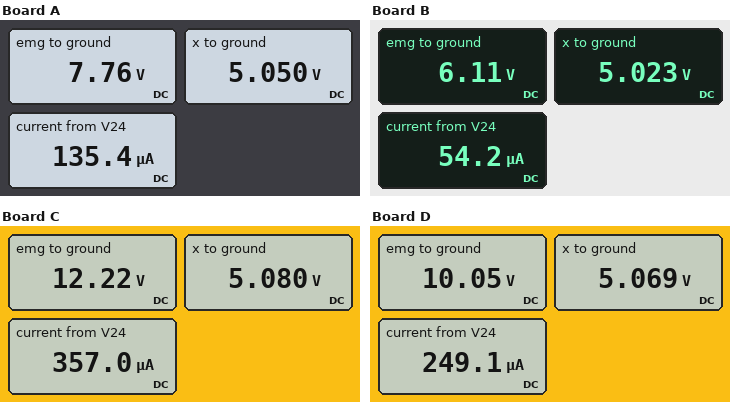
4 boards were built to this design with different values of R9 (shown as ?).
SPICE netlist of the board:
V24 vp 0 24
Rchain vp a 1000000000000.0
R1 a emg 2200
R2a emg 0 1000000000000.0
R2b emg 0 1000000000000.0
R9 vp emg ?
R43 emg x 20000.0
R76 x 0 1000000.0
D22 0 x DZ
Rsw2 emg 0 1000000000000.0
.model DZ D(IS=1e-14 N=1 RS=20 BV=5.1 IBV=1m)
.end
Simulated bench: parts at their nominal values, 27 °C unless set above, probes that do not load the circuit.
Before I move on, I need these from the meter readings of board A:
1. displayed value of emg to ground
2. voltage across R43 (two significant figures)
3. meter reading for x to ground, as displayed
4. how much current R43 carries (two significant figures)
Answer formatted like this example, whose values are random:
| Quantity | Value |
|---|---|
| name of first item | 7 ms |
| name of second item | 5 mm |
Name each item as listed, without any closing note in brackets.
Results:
| Quantity | Value |
|---|---|
| displayed value of emg to ground | 7.76 V |
| voltage across R43 | 2.7 V |
| meter reading for x to ground, as displayed | 5.050 V |
| how much current R43 carries | 140 µA |
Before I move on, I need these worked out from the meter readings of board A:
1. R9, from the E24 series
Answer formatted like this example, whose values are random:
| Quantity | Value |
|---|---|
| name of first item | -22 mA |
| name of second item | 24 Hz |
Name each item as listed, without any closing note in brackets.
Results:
| Quantity | Value |
|---|---|
| R9, from the E24 series | 120 kΩ |
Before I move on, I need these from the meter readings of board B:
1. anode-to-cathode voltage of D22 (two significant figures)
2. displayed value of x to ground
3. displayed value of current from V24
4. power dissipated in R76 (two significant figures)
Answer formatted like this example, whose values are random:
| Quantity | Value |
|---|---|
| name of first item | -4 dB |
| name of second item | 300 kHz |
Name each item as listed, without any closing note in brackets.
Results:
| Quantity | Value |
|---|---|
| anode-to-cathode voltage of D22 | -5.0 V |
| displayed value of x to ground | 5.023 V |
| displayed value of current from V24 | 54.2 µA |
| power dissipated in R76 | 25 µW |
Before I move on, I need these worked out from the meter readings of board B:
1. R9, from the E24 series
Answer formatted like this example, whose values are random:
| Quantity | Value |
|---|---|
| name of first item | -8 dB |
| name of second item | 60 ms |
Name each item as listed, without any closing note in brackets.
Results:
| Quantity | Value |
|---|---|
| R9, from the E24 series | 330 kΩ |
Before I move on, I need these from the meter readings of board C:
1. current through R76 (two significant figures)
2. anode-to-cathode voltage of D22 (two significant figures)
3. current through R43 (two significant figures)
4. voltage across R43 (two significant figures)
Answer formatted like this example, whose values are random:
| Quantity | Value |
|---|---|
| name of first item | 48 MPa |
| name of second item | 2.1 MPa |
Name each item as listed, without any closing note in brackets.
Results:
| Quantity | Value |
|---|---|
| current through R76 | 5.1 µA |
| anode-to-cathode voltage of D22 | -5.1 V |
| current through R43 | 360 µA |
| voltage across R43 | 7.1 V |
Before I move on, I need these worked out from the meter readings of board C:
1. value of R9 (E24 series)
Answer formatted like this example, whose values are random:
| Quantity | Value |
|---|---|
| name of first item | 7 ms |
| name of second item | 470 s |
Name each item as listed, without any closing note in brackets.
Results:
| Quantity | Value |
|---|---|
| value of R9 | 33 kΩ |
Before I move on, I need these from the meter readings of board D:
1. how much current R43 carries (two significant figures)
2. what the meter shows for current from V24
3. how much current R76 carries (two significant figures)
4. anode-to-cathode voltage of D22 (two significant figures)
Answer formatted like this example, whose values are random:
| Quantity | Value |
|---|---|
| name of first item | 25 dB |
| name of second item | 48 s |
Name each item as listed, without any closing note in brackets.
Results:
| Quantity | Value |
|---|---|
| how much current R43 carries | 250 µA |
| what the meter shows for current from V24 | 249.1 µA |
| how much current R76 carries | 5.1 µA |
| anode-to-cathode voltage of D22 | -5.1 V |
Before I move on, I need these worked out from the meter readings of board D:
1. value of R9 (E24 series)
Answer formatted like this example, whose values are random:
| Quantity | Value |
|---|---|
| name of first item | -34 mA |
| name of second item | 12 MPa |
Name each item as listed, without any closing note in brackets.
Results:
| Quantity | Value |
|---|---|
| value of R9 | 56 kΩ |
